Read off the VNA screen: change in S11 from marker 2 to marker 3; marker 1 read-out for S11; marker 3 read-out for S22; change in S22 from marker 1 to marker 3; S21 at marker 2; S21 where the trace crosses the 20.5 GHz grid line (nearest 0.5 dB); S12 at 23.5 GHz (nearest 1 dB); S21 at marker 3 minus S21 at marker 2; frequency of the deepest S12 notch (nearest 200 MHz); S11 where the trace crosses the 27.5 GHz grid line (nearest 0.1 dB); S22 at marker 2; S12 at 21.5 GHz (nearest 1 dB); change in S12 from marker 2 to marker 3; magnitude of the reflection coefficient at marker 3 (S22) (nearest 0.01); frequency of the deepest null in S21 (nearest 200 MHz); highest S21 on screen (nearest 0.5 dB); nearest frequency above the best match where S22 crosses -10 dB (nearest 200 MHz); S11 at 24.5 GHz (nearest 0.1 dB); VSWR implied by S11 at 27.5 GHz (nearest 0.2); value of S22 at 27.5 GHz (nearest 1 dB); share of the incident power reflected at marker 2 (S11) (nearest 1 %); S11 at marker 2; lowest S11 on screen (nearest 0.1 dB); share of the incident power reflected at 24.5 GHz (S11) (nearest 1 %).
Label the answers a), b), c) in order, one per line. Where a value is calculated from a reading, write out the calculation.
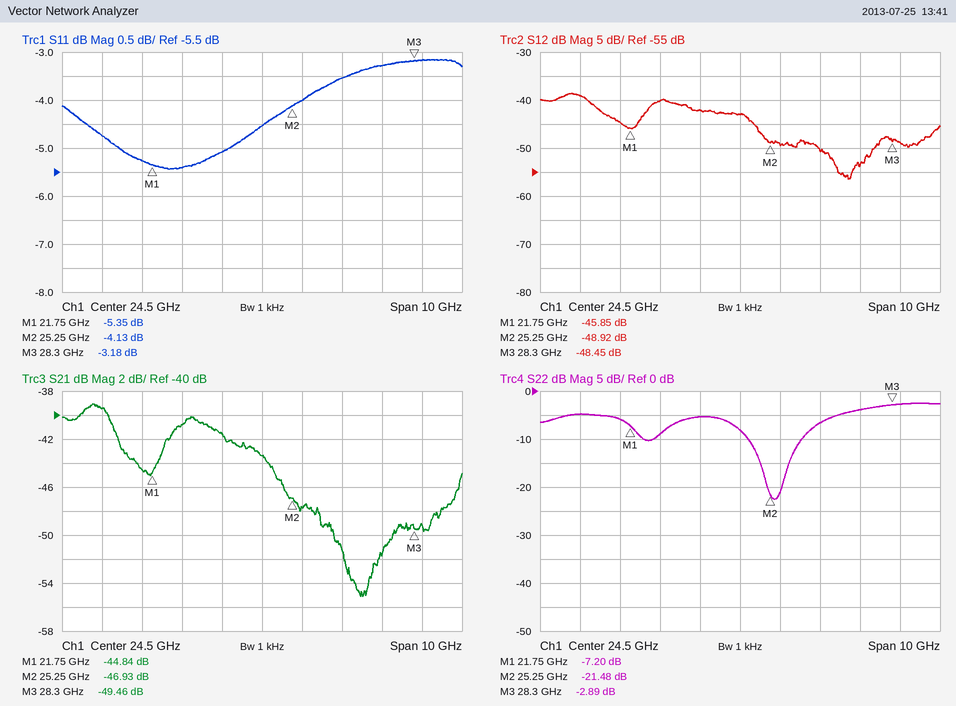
a) -3.18 − (-4.13) = 0.95 dB
b) -5.35 dB
c) -2.89 dB
d) -2.89 − (-7.2) = 4.31 dB
e) -46.93 dB
f) -39.5 dB
g) -42 dB
h) -49.46 − (-46.93) = -2.53 dB
i) 27.2 GHz
j) -3.3 dB
k) -21.48 dB
l) -45 dB
m) -48.45 − (-48.92) = 0.47 dB
n) 10^(-2.89/20) ≈ 0.72
o) 27.0 GHz
p) -39.0 dB
q) 26.0 GHz
r) -4.5 dB
s) |Γ| = 10^(-3.3/20) = 0.6839; VSWR = (1 + 0.6839)/(1 − 0.6839) ≈ 5.33, so 5.4 to the nearest 0.2
t) -4 dB
u) 10^(-4.13/10) ≈ 39 %
v) -4.13 dB
w) -5.4 dB
x) 10^(-4.5/10) ≈ 35 %
